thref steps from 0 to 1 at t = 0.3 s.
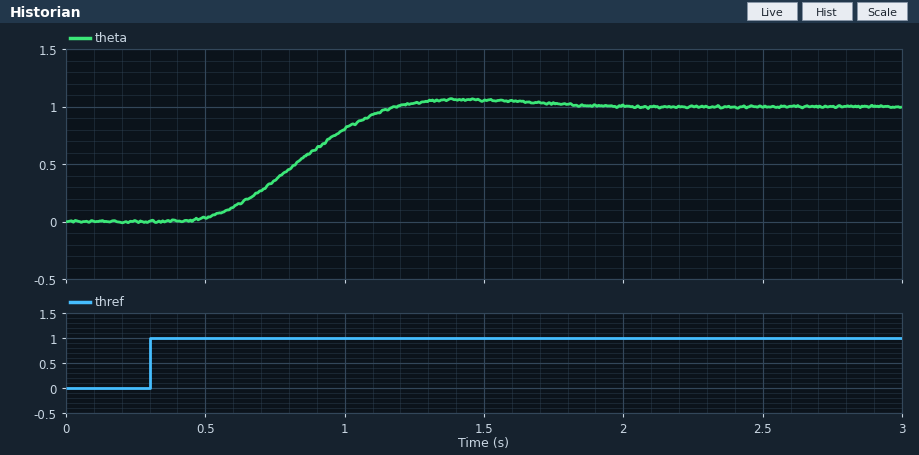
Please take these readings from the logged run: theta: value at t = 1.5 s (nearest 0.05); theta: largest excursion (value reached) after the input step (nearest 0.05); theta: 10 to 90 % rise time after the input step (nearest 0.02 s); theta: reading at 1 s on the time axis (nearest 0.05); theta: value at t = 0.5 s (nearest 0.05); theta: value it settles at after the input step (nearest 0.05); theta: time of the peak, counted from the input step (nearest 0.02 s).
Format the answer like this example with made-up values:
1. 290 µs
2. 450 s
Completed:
1. 1.05
2. 1.05
3. 0.50 s
4. 0.80
5. 0.05
6. 1.00
7. 1.12 s
